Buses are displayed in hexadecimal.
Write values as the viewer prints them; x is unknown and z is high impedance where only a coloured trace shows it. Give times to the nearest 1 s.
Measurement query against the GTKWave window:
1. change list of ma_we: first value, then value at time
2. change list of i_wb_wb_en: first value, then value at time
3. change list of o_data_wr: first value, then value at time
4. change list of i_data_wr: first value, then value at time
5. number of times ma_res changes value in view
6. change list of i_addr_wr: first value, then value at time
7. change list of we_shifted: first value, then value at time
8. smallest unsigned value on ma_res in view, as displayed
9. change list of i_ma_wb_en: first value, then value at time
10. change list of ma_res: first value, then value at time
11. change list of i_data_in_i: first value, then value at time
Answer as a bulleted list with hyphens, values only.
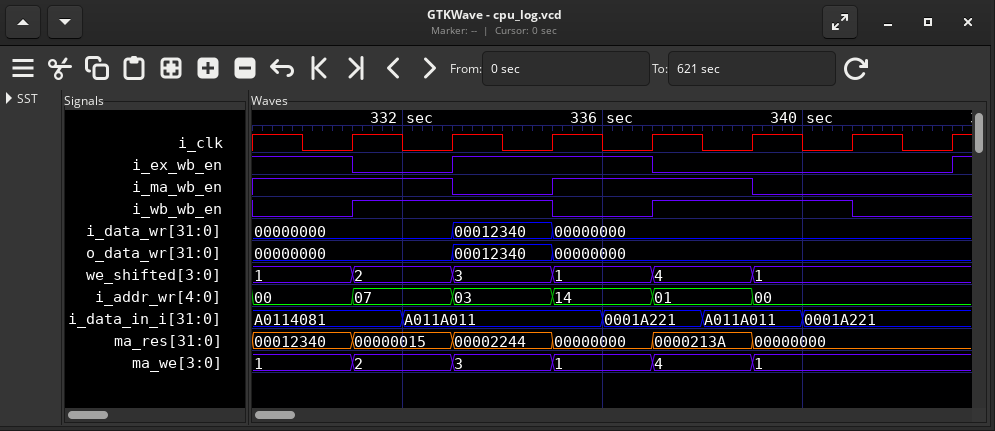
- 1, 2 at 331 s, 3 at 333 s, 1 at 335 s, 4 at 337 s, 1 at 339 s
- 0, 1 at 331 s, 0 at 335 s, 1 at 337 s, 0 at 341 s
- 00000000, 00012340 at 333 s, 00000000 at 335 s
- 00000000, 00012340 at 333 s, 00000000 at 335 s
- 5
- 00, 07 at 331 s, 03 at 333 s, 14 at 335 s, 01 at 337 s, 00 at 339 s
- 1, 2 at 331 s, 3 at 333 s, 1 at 335 s, 4 at 337 s, 1 at 339 s
- 00000000
- 1, 0 at 333 s, 1 at 335 s, 0 at 339 s
- 00012340, 00000015 at 331 s, 00002244 at 333 s, 00000000 at 335 s, 0000213A at 337 s, 00000000 at 339 s
- A0114081, A011A011 at 332 s, 0001A221 at 336 s, A011A011 at 338 s, 0001A221 at 340 s
